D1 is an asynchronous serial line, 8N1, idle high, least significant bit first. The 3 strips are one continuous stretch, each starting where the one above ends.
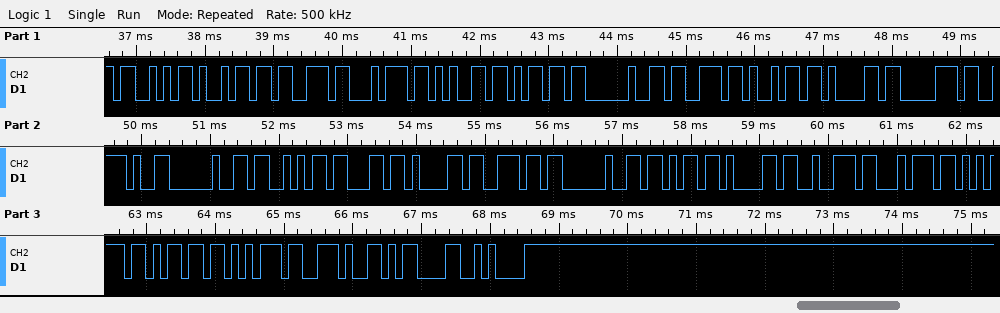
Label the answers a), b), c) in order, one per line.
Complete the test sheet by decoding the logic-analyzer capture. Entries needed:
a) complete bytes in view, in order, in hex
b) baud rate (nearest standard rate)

a) 53 69 73 74 65 6D 20 73 69 61 70 2E 20 53 63 61 6E 20 6B 61 72 74 75 6D 75 2E 0D 0A
b) 9600 baud
